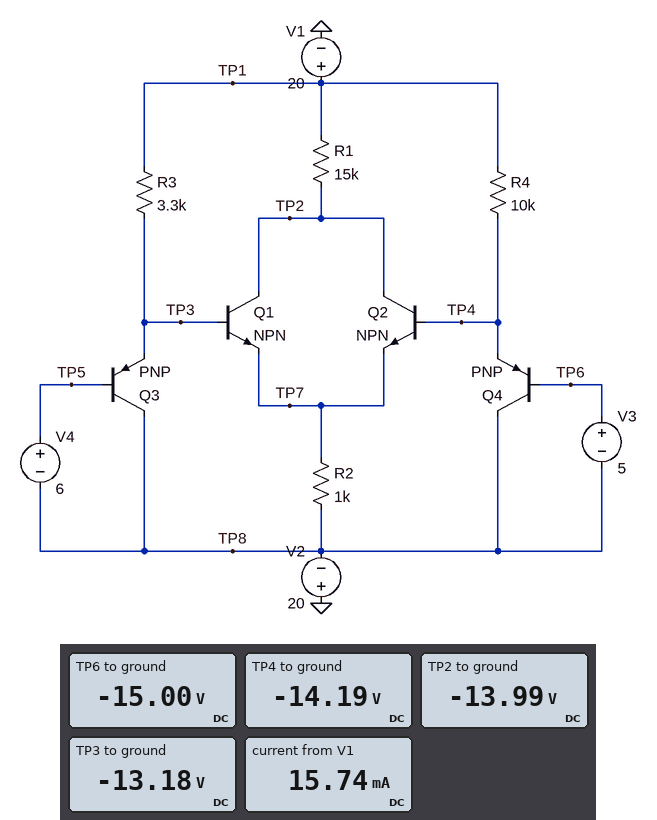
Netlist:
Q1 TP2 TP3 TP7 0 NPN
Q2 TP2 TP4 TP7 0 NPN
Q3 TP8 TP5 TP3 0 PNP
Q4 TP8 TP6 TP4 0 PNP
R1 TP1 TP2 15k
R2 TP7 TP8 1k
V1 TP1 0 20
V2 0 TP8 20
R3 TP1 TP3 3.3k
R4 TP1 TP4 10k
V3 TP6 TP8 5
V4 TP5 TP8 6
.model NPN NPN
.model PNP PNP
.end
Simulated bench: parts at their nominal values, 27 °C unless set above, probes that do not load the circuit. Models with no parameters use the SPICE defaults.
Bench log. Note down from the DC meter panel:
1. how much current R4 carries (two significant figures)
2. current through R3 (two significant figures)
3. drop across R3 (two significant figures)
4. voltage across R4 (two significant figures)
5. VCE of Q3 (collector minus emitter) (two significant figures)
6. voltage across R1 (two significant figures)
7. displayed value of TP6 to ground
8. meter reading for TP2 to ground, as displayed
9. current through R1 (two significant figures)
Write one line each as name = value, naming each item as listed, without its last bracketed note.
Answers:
how much current R4 carries = 3.4 mA
current through R3 = 10 mA
drop across R3 = 33 V
voltage across R4 = 34 V
VCE of Q3 (collector minus emitter) = -6.8 V
voltage across R1 = 34 V
displayed value of TP6 to ground = -15.00 V
meter reading for TP2 to ground, as displayed = -13.99 V
current through R1 = 2.3 mA
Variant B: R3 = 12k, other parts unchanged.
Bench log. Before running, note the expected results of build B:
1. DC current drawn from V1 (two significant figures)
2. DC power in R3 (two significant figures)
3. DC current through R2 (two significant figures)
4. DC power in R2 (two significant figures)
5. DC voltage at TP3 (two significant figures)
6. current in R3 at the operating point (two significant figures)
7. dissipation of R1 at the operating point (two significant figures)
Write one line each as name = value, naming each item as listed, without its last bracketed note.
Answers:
DC current drawn from V1 = 8.6 mA
DC power in R3 = 96 mW
DC current through R2 = 5.2 mA
DC power in R2 = 27 mW
DC voltage at TP3 = -14 V
current in R3 at the operating point = 2.8 mA
dissipation of R1 at the operating point = 81 mW
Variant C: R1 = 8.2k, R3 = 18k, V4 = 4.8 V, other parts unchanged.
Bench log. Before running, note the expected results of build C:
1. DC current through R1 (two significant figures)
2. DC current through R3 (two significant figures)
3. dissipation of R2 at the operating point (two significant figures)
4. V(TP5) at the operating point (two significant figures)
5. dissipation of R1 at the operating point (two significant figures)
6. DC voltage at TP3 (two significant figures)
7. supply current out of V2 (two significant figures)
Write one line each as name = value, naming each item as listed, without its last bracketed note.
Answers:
DC current through R1 = 4.3 mA
DC current through R3 = 1.9 mA
dissipation of R2 at the operating point = 25 mW
V(TP5) at the operating point = -15 V
dissipation of R1 at the operating point = 150 mW
DC voltage at TP3 = -14 V
supply current out of V2 = 9.6 mA
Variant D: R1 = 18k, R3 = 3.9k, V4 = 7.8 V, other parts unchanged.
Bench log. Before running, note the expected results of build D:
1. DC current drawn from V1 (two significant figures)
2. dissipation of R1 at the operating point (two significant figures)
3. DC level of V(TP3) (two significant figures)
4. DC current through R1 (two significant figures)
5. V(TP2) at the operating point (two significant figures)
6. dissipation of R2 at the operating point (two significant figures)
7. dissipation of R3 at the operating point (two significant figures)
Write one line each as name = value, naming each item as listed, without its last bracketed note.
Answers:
DC current drawn from V1 = 13 mA
dissipation of R1 at the operating point = 58 mW
DC level of V(TP3) = -11 V
DC current through R1 = 1.8 mA
V(TP2) at the operating point = -12 V
dissipation of R2 at the operating point = 60 mW
dissipation of R3 at the operating point = 250 mW
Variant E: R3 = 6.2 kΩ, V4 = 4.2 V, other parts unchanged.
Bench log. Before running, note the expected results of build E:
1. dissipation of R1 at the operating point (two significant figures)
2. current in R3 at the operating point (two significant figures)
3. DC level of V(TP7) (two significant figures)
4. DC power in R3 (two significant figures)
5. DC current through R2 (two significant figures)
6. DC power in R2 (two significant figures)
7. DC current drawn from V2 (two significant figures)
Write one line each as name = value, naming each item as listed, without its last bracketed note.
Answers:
dissipation of R1 at the operating point = 82 mW
current in R3 at the operating point = 5.6 mA
DC level of V(TP7) = -15 V
DC power in R3 = 200 mW
DC current through R2 = 4.9 mA
DC power in R2 = 24 mW
DC current drawn from V2 = 11 mA
